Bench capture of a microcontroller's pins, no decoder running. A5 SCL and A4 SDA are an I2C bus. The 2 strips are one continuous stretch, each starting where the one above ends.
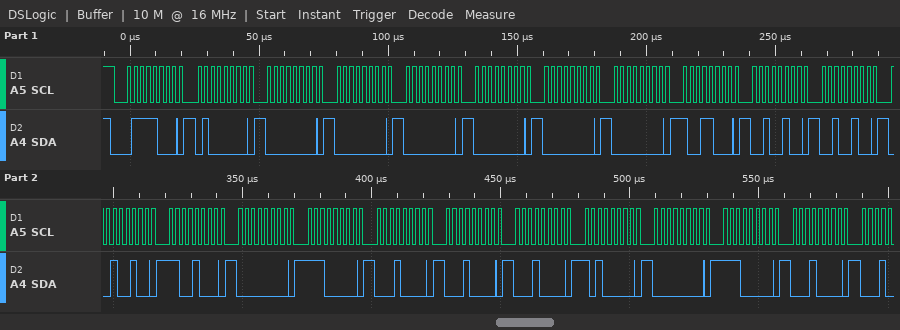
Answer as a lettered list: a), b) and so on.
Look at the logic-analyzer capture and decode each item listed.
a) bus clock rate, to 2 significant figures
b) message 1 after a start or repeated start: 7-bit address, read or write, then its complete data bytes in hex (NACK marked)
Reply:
a) 400 kHz
b) 0x3C write: 40 00 00 00 00 00 00 98 24 24 24 C8 00 E0 10 10 10 A0 00 E0 10
